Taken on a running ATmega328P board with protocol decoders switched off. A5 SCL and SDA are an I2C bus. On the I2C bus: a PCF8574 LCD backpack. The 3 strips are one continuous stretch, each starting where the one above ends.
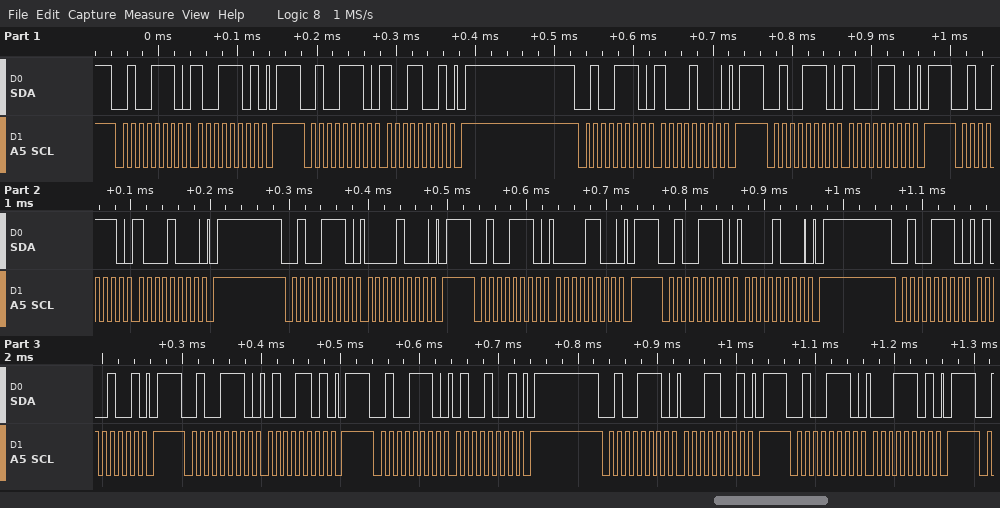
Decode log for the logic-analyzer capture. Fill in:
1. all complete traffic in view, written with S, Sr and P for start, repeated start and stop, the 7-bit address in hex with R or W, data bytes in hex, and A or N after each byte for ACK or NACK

S 27W A 9D A P S 27W A 99 A P S 27W A 88 A P S 27W A 8C A P S 27W A 88 A P S 27W A 08 A P S 27W A 0C A P S 27W A 08 A P S 27W A 49 A P S 27W A 4D A P S 27W A 49 A P S 27W A 19 A P S 27W A 1D A P
